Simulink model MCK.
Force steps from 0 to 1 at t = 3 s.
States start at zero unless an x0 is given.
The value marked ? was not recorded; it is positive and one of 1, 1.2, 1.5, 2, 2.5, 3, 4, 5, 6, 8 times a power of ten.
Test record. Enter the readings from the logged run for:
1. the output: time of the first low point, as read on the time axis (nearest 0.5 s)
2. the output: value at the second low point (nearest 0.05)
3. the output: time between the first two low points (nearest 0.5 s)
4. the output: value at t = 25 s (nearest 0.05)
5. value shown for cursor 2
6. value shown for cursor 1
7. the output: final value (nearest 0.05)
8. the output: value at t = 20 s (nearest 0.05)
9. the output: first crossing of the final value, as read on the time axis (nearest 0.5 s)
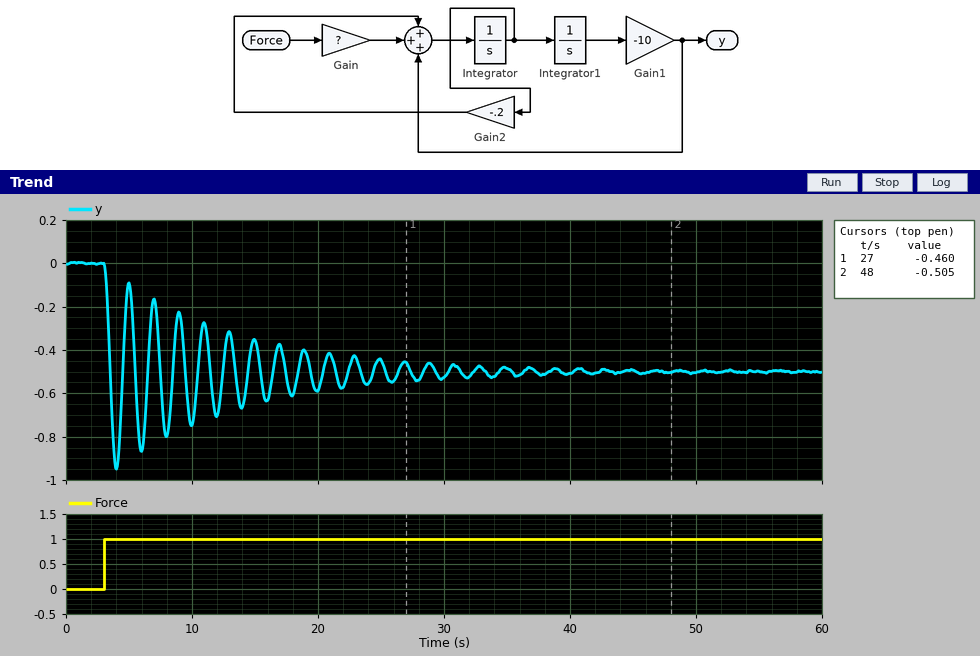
4.0 s
-0.85
2.0 s
-0.45
-0.505
-0.460
-0.50
-0.60
3.5 s
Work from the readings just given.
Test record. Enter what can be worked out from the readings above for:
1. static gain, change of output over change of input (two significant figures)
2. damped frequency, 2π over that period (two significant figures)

-0.50
3.1 rad/s
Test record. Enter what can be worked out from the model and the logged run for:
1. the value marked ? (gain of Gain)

0.5
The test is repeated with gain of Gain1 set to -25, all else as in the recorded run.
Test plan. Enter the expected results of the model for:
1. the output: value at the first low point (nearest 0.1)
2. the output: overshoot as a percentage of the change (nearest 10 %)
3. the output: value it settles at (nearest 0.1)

-1.0
90 %
-0.5
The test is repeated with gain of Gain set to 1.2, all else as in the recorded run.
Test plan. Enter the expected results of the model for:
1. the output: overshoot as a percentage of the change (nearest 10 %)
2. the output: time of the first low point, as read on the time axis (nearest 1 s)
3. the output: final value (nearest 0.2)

90 %
4 s
-1.2
